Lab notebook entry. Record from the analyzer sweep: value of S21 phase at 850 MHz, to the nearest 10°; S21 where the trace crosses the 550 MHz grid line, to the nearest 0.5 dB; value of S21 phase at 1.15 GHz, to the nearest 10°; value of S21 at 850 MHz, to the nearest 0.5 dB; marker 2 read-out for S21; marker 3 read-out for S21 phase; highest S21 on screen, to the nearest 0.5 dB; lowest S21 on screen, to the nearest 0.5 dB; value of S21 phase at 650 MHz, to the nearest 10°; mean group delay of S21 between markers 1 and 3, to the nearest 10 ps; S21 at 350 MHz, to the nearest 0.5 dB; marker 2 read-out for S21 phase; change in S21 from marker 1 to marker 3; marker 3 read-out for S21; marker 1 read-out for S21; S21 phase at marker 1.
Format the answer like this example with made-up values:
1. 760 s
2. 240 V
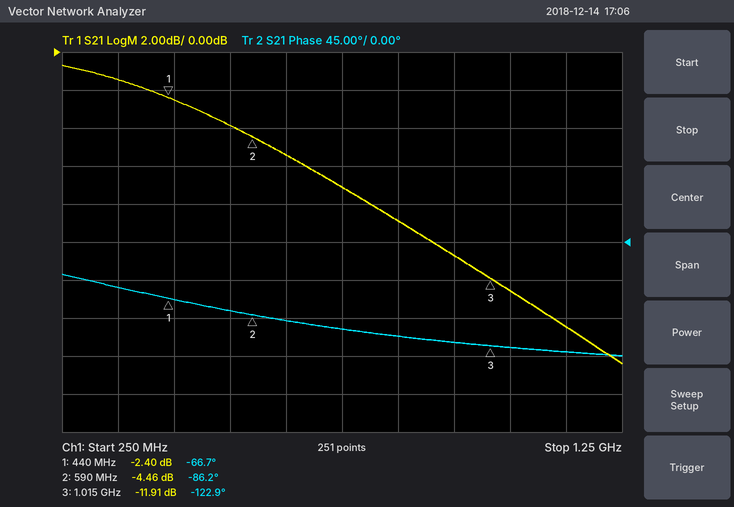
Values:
1. -110°
2. -4.0 dB
3. -130°
4. -9.0 dB
5. -4.46 dB
6. -122.9°
7. -0.5 dB
8. -16.5 dB
9. -90°
10. 270 ps
11. -1.5 dB
12. -86.2°
13. -9.51 dB
14. -11.91 dB
15. -2.40 dB
16. -66.7°
